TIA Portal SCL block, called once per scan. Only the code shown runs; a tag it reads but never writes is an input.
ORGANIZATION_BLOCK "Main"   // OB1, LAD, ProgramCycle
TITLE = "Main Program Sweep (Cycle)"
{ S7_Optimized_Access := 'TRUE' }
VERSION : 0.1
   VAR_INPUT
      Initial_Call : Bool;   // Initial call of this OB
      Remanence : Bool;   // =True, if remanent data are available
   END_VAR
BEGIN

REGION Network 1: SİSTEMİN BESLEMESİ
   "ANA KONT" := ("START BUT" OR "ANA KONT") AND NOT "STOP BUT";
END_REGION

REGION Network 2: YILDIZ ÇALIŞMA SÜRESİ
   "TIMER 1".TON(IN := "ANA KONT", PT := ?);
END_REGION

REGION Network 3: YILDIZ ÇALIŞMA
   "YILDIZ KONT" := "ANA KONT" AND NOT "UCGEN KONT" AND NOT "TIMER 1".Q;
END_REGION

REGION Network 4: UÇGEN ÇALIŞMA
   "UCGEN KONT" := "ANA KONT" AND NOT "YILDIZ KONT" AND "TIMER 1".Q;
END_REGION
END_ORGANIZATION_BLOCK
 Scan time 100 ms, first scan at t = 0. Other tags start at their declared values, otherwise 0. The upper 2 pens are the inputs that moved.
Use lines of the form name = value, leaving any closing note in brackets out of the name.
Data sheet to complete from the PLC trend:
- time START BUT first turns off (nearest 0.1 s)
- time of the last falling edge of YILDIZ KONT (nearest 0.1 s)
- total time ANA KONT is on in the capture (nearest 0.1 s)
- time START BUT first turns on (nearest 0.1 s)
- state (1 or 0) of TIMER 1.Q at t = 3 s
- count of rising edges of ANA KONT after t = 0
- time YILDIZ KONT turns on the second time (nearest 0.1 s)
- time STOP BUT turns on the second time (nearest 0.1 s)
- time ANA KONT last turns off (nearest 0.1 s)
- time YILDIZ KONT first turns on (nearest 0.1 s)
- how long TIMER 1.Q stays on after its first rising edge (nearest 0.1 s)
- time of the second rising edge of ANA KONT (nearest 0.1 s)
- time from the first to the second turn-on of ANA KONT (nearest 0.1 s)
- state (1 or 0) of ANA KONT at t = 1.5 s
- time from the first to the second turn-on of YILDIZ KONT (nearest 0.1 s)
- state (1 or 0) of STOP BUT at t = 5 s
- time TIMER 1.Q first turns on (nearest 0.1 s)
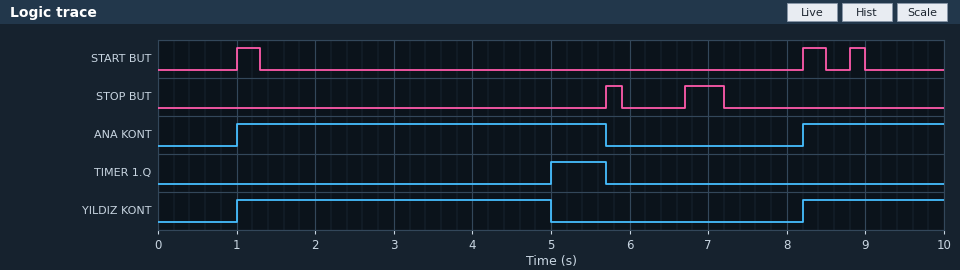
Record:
time START BUT first turns off = 1.3 s
time of the last falling edge of YILDIZ KONT = 5.0 s
total time ANA KONT is on in the capture = 6.5 s
time START BUT first turns on = 1.0 s
state (1 or 0) of TIMER 1.Q at t = 3 s = 0
count of rising edges of ANA KONT after t = 0 = 2
time YILDIZ KONT turns on the second time = 8.2 s
time STOP BUT turns on the second time = 6.7 s
time ANA KONT last turns off = 5.7 s
time YILDIZ KONT first turns on = 1.0 s
how long TIMER 1.Q stays on after its first rising edge = 0.7 s
time of the second rising edge of ANA KONT = 8.2 s
time from the first to the second turn-on of ANA KONT = 7.2 s
state (1 or 0) of ANA KONT at t = 1.5 s = 1
time from the first to the second turn-on of YILDIZ KONT = 7.2 s
state (1 or 0) of STOP BUT at t = 5 s = 0
time TIMER 1.Q first turns on = 5.0 s
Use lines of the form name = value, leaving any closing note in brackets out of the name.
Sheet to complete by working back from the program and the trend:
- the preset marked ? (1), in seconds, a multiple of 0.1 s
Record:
the preset marked ? (1), in seconds, a multiple of 0.1 s = 4.0 s
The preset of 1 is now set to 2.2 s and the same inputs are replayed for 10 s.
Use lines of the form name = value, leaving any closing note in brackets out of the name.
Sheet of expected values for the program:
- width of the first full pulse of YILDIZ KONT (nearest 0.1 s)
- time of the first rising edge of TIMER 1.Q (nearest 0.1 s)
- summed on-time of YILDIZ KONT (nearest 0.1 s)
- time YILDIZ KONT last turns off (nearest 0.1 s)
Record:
width of the first full pulse of YILDIZ KONT = 2.2 s
time of the first rising edge of TIMER 1.Q = 3.2 s
summed on-time of YILDIZ KONT = 4.0 s
time YILDIZ KONT last turns off = 3.2 s
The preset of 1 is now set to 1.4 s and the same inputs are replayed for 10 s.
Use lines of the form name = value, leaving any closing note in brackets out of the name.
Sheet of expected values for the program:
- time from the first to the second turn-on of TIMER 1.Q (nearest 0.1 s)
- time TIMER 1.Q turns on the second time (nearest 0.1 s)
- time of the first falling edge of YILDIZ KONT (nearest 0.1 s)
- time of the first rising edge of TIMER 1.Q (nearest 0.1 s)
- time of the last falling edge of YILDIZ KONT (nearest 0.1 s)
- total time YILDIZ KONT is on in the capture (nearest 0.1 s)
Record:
time from the first to the second turn-on of TIMER 1.Q = 7.2 s
time TIMER 1.Q turns on the second time = 9.6 s
time of the first falling edge of YILDIZ KONT = 2.4 s
time of the first rising edge of TIMER 1.Q = 2.4 s
time of the last falling edge of YILDIZ KONT = 9.6 s
total time YILDIZ KONT is on in the capture = 2.8 s
